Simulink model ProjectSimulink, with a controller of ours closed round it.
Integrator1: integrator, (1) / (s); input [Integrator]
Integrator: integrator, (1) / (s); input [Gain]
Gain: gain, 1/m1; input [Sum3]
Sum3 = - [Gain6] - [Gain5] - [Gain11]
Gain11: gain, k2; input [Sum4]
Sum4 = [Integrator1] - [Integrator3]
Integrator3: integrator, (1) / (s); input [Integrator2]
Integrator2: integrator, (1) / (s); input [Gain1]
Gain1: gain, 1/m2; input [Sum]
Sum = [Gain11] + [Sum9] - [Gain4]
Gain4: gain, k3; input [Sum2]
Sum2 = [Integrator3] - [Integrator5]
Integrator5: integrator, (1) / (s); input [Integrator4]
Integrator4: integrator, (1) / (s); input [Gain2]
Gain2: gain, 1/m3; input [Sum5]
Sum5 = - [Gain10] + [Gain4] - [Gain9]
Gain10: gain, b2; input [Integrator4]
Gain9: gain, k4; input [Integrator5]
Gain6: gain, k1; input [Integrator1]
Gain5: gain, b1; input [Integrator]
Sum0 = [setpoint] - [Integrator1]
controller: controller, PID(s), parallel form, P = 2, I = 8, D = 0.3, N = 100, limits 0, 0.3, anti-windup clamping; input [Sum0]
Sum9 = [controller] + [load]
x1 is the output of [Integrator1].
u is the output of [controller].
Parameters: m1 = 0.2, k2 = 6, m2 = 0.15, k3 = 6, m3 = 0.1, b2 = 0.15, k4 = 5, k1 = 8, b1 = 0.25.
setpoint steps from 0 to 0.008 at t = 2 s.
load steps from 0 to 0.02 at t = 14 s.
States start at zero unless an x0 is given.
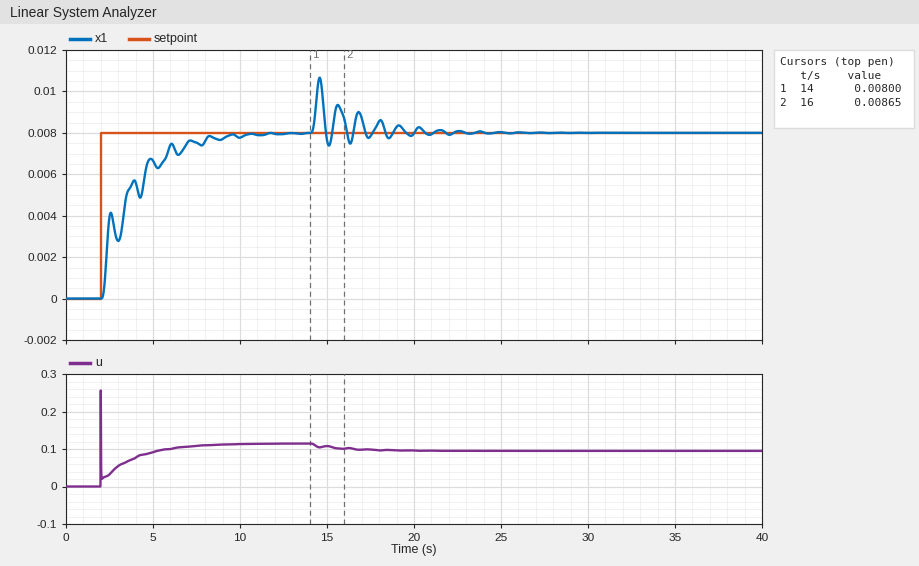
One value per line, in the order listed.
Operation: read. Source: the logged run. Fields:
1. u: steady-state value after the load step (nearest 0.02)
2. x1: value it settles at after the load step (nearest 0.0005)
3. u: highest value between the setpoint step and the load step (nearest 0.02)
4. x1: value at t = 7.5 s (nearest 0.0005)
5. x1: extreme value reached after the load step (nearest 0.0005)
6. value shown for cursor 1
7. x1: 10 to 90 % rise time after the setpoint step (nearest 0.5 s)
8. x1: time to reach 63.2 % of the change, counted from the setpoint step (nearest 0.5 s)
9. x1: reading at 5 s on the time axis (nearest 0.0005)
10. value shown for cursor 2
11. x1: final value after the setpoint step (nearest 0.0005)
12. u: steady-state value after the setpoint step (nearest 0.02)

0.10
0.0080
0.26
0.0075
0.0105
0.00800
3.5 s
1.5 s
0.0065
0.00865
0.0080
0.12
